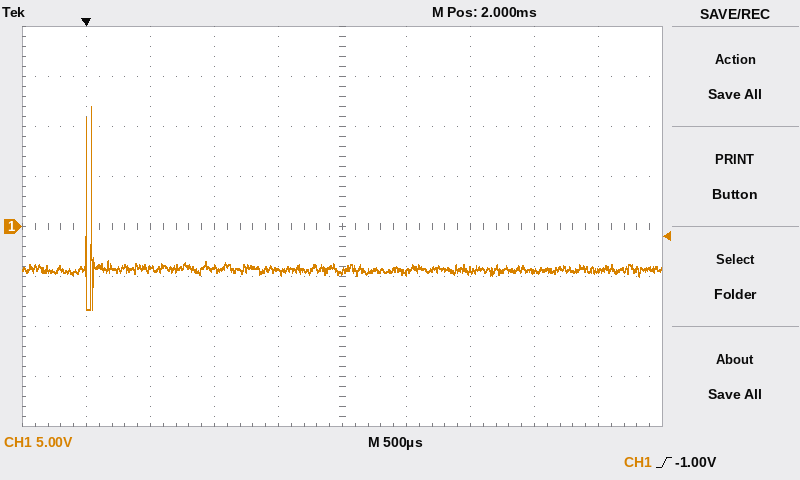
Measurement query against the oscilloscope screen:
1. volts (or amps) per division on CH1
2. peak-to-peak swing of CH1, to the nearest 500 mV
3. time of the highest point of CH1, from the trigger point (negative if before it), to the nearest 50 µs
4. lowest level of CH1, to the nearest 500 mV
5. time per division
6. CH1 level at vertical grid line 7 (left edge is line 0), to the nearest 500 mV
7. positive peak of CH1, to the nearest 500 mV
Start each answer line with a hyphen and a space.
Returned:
- 5 V
- 20.5 V
- +50 µs
- -8.5 V
- 500 µs
- -4.5 V
- 12.0 V
